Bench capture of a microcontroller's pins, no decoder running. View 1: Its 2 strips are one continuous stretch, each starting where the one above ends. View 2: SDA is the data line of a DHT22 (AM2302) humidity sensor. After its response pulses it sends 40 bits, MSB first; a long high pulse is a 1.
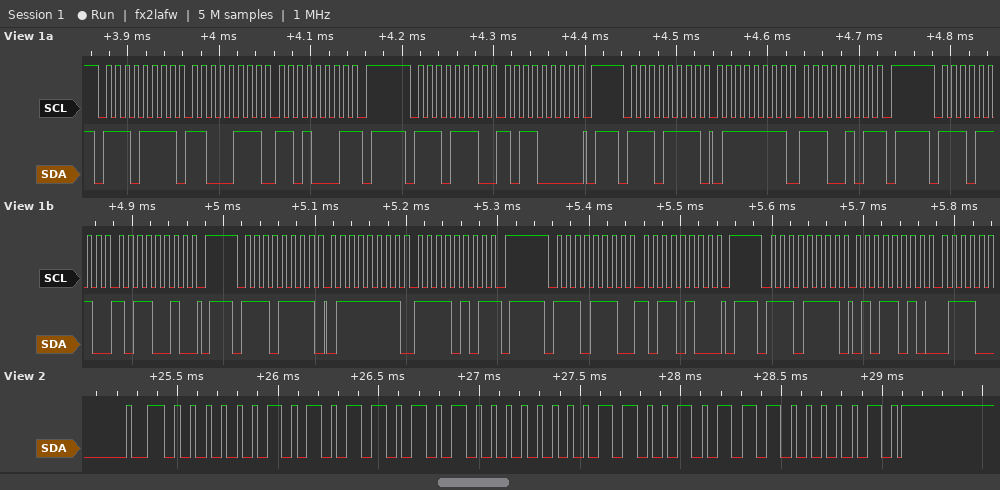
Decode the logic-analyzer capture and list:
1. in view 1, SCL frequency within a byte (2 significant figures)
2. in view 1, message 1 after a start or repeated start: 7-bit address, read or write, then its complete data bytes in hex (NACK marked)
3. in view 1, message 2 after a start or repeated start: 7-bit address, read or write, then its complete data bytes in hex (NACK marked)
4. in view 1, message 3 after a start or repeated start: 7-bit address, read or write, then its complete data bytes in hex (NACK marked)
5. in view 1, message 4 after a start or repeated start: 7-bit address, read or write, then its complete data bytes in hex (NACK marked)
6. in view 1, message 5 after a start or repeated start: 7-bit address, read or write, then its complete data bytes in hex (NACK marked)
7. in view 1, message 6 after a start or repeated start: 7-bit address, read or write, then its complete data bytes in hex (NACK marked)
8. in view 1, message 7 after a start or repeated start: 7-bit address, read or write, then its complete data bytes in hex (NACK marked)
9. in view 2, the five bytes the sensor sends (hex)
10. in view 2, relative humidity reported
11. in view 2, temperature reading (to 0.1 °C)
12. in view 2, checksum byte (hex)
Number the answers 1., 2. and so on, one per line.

1. 100 kHz
2. 0x77 read: C7 D1 NACK
3. 0x77 write: B0
4. 0x77 read: 7F E5 NACK
5. 0x77 write: B2
6. 0x77 read: 7F F5 NACK
7. 0x77 write: B4
8. 0x77 read: 5A
9. 02 B5 00 CB 82
10. 69.3 %
11. 20.3 °C
12. 0x82
